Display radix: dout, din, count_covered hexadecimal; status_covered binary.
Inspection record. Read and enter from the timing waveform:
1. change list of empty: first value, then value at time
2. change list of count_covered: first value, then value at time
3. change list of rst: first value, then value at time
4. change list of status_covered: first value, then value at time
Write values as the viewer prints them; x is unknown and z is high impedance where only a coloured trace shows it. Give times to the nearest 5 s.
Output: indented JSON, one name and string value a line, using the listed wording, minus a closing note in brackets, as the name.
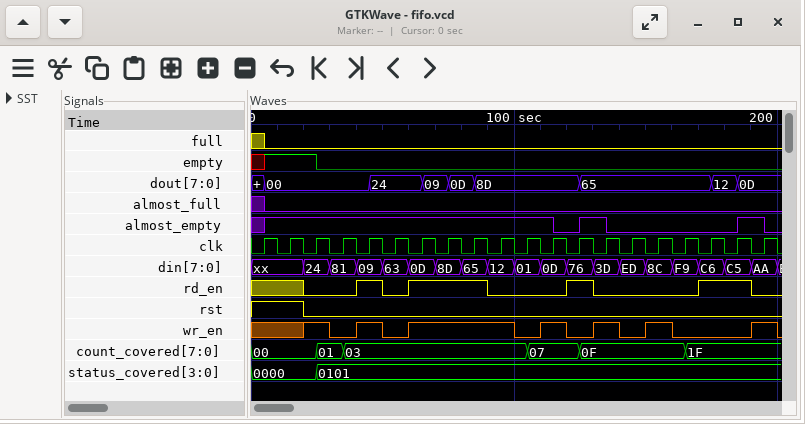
{
  "change list of empty: first value, then value at time": "x, 1 at 5 s, 0 at 25 s",
  "change list of count_covered: first value, then value at time": "00, 01 at 25 s, 03 at 35 s, 07 at 105 s, 0F at 125 s, 1F at 165 s",
  "change list of rst: first value, then value at time": "1, 0 at 20 s",
  "change list of status_covered: first value, then value at time": "0000, 0101 at 25 s"
}
